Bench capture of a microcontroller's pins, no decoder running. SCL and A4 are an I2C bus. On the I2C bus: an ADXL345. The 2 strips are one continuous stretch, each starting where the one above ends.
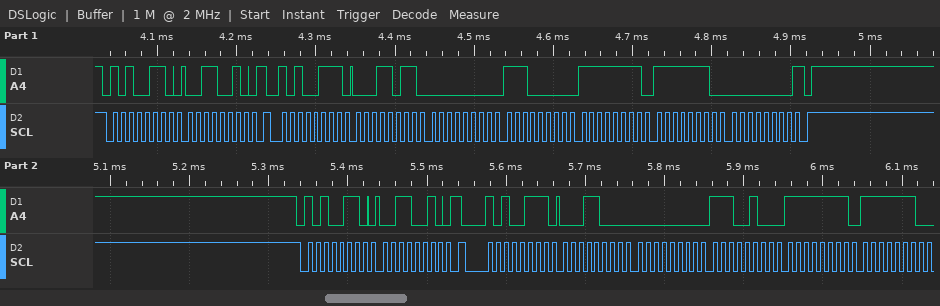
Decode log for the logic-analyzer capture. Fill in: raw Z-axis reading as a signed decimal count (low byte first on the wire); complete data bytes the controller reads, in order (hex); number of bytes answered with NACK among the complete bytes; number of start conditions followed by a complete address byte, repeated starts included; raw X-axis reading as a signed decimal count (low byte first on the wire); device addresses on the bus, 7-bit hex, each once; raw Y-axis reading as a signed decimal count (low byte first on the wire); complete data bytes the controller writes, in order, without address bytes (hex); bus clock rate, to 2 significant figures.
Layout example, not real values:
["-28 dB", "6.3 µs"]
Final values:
["254", "1B 00 E0 FF FE 00 18 00 E4 FF FE", "1", "4", "27", "0x53", "-32", "32 32", "100 kHz"]
